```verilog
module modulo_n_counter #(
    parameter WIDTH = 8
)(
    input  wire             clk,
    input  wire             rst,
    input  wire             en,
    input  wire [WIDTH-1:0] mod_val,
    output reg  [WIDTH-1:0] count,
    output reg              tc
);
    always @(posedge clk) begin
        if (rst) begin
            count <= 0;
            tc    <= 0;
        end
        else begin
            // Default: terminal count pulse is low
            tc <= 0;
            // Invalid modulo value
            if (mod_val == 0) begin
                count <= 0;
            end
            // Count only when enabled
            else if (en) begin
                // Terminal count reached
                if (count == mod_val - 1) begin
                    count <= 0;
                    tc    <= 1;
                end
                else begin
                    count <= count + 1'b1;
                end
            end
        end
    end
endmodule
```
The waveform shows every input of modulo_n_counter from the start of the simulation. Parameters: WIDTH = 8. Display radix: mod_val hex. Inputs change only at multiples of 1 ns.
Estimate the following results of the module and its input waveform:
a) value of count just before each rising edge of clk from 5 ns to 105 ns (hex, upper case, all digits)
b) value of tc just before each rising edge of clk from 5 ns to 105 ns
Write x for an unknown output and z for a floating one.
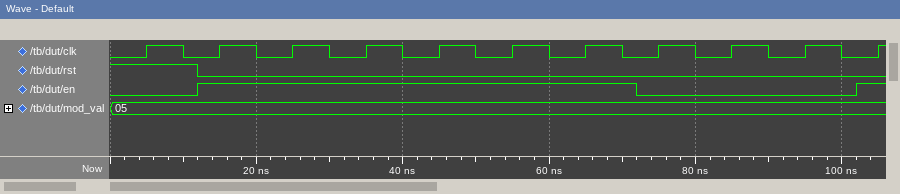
x, 00, 01, 02, 03, 04, 00, 01, 01, 01, 01
x 0 0 0 0 0 1 0 0 0 0
